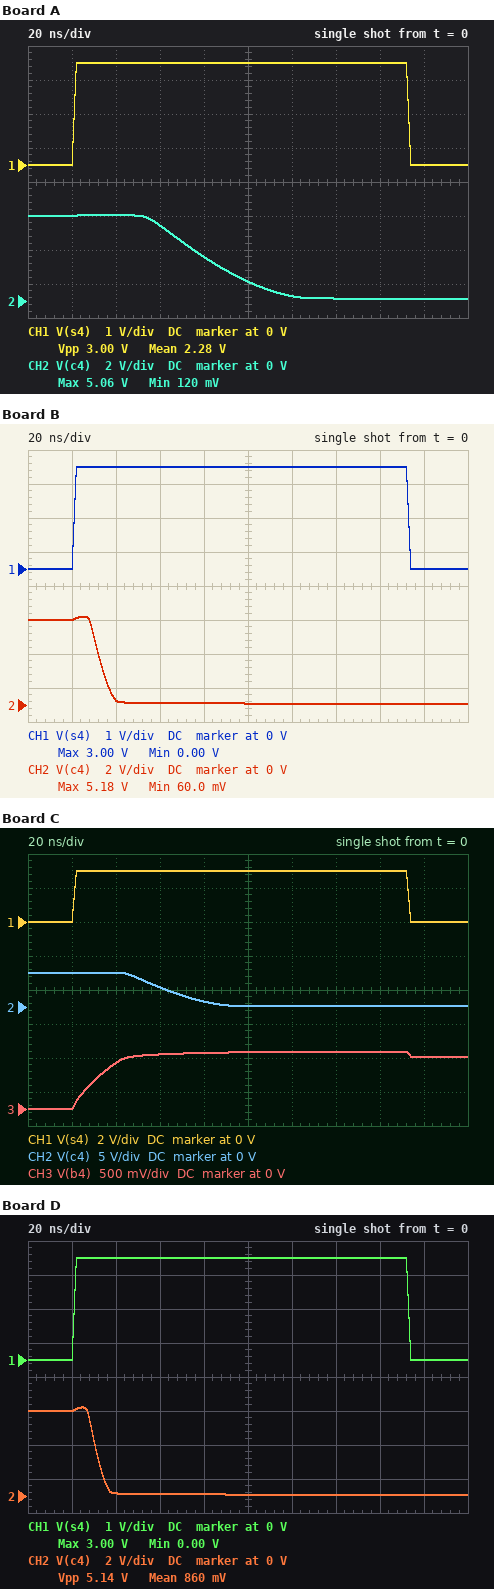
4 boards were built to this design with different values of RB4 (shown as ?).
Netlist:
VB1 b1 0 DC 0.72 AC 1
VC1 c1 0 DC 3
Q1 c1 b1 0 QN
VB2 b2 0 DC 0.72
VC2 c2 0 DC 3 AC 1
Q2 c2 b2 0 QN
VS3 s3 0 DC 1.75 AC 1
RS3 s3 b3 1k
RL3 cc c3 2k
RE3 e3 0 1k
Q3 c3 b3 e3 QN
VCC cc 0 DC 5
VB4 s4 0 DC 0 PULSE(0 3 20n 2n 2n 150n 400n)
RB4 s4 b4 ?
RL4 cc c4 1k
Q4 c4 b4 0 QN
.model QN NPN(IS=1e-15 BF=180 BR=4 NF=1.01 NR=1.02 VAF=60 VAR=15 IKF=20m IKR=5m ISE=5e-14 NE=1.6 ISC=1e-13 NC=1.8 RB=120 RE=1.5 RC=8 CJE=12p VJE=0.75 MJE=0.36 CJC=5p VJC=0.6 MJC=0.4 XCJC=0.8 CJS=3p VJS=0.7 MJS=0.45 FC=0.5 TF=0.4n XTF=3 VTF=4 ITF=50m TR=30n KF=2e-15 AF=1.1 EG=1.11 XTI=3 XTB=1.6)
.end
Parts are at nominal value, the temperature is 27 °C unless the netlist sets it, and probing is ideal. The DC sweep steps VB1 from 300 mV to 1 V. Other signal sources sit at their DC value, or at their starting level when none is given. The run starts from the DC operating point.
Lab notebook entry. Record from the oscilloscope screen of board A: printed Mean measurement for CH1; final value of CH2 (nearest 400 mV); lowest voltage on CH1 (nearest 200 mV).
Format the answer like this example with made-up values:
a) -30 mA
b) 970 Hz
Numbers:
a) 2.28 V
b) 0 V
c) 0 V
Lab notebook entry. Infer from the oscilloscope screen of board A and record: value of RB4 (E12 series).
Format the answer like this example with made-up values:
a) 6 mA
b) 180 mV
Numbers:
a) 6.8 kΩ
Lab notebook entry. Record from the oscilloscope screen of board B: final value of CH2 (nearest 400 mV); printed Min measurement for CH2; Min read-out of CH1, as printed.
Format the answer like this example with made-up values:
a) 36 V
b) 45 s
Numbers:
a) 0 V
b) 60.0 mV
c) 0.00 V
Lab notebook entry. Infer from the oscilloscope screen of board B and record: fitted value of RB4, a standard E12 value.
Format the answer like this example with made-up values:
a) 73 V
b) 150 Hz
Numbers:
a) 1.2 kΩ
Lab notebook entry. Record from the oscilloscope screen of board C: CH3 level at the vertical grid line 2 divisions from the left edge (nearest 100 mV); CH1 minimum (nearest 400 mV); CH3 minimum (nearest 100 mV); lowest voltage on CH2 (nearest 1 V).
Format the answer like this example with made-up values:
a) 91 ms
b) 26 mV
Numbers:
a) 700 mV
b) 0 V
c) 0 V
d) 0 V
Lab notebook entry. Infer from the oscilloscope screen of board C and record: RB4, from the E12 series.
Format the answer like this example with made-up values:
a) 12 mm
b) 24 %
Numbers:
a) 4.7 kΩ
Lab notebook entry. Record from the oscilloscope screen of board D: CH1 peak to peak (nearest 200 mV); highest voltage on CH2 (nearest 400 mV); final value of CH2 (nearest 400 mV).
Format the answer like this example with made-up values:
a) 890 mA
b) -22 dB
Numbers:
a) 3.0 V
b) 5.2 V
c) 0 V
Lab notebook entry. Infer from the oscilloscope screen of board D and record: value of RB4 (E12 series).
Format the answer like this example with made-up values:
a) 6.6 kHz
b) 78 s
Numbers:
a) 1 kΩ
